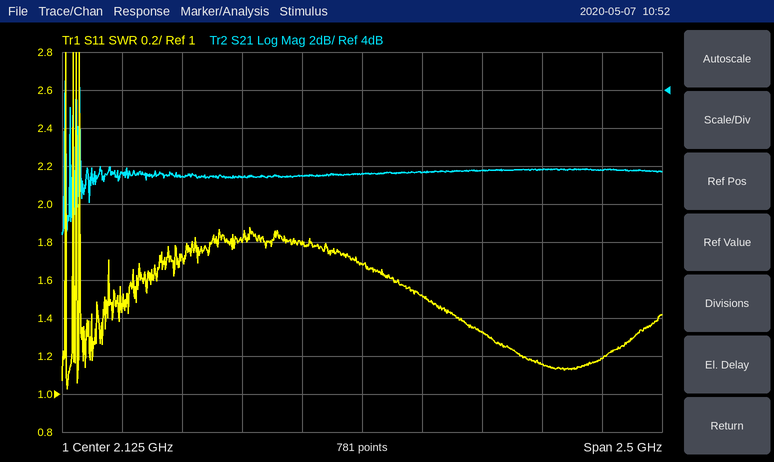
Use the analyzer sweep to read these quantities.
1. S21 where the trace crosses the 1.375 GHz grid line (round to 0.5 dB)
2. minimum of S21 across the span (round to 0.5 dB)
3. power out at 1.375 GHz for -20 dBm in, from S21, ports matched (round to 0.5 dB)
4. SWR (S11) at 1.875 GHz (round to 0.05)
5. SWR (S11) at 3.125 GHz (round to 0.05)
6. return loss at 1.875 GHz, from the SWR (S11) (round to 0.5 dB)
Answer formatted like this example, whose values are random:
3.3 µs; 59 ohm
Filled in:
-0.5 dB; -3.5 dB; -20.5 dBm; 1.80; 1.20; 11.0 dB
